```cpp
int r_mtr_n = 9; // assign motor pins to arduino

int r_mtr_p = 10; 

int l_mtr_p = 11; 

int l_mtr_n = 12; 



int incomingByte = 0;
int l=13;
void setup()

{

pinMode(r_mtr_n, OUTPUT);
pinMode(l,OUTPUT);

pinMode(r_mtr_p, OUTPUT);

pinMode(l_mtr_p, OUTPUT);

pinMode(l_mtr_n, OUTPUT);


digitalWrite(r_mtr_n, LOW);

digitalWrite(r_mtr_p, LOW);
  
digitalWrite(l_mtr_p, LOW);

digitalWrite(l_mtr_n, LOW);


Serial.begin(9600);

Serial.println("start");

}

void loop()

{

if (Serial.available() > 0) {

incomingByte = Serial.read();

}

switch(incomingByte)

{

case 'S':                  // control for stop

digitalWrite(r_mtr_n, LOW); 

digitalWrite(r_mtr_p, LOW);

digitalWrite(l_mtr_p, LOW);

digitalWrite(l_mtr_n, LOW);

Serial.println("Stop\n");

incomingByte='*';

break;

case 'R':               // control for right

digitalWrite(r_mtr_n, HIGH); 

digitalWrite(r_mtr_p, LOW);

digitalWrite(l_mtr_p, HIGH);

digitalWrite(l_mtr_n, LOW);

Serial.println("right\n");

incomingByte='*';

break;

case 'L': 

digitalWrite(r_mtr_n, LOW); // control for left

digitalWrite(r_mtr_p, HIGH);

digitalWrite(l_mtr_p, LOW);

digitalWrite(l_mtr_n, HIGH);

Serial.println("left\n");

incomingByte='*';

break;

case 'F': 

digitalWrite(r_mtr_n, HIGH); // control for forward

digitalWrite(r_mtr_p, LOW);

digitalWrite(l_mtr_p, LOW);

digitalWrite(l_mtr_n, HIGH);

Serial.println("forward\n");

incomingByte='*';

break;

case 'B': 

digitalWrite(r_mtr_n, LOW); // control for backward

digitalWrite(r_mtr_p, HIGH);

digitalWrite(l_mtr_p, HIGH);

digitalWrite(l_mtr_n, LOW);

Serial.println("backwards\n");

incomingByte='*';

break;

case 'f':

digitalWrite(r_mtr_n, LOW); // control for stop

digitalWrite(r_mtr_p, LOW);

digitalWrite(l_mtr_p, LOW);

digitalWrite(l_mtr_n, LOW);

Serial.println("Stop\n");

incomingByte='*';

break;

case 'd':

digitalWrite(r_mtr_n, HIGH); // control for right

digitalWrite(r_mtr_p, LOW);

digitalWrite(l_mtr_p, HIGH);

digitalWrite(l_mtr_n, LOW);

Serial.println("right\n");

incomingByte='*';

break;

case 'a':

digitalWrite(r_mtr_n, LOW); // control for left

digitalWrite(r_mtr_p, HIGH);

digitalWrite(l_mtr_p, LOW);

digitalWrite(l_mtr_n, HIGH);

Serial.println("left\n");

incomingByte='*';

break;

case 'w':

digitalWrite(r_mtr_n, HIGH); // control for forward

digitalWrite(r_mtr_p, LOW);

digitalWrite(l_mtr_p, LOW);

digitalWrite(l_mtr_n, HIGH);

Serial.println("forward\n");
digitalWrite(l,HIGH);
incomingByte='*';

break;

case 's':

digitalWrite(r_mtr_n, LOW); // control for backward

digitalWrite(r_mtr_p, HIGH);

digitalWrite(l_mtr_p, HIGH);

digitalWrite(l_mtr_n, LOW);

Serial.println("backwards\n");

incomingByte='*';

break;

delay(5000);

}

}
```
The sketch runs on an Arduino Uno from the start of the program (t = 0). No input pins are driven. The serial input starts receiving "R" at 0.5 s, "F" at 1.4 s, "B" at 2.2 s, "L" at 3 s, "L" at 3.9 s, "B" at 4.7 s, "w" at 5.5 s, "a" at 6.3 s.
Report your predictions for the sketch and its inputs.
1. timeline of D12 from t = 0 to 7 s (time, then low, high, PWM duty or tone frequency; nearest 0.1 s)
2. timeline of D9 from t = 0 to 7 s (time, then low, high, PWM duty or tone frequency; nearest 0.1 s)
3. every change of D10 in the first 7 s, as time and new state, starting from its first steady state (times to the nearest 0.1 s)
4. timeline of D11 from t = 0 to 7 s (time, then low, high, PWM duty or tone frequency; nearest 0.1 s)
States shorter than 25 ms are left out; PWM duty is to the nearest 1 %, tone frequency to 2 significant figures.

0 s low; 1.4 s high; 2.2 s low; 3 s high; 4.7 s low; 5.5 s high
0 s low; 0.5 s high; 2.2 s low; 5.5 s high; 6.3 s low
0 s low; 2.2 s high; 5.5 s low; 6.3 s high
0 s low; 0.5 s high; 1.4 s low; 2.2 s high; 3 s low; 4.7 s high; 5.5 s low
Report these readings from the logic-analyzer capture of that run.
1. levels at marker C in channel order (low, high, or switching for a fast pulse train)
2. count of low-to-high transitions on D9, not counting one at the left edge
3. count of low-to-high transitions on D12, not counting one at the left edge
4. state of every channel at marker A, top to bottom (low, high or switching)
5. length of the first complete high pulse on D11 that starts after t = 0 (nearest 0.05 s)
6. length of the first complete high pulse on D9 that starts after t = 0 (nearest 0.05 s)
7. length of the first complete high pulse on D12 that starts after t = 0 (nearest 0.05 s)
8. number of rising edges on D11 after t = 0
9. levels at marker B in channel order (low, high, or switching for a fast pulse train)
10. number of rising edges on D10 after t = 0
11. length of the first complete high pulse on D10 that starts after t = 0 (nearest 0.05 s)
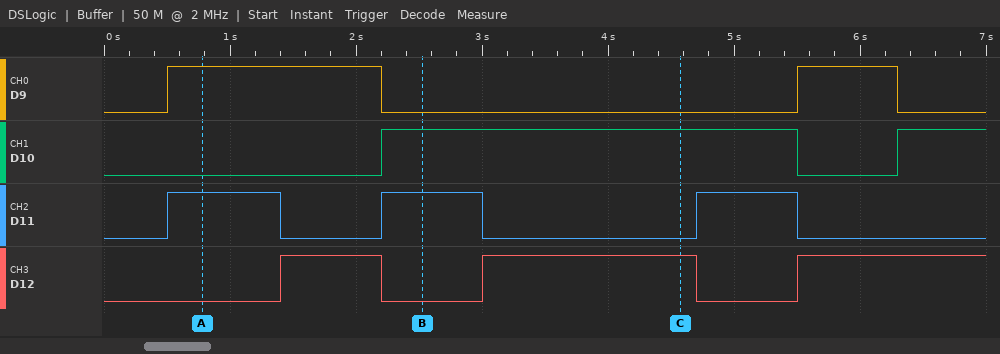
D9 low, D10 high, D11 low, D12 high
2
3
D9 high, D10 low, D11 high, D12 low
0.90 s
1.70 s
0.80 s
3
D9 low, D10 high, D11 high, D12 low
2
3.30 s
